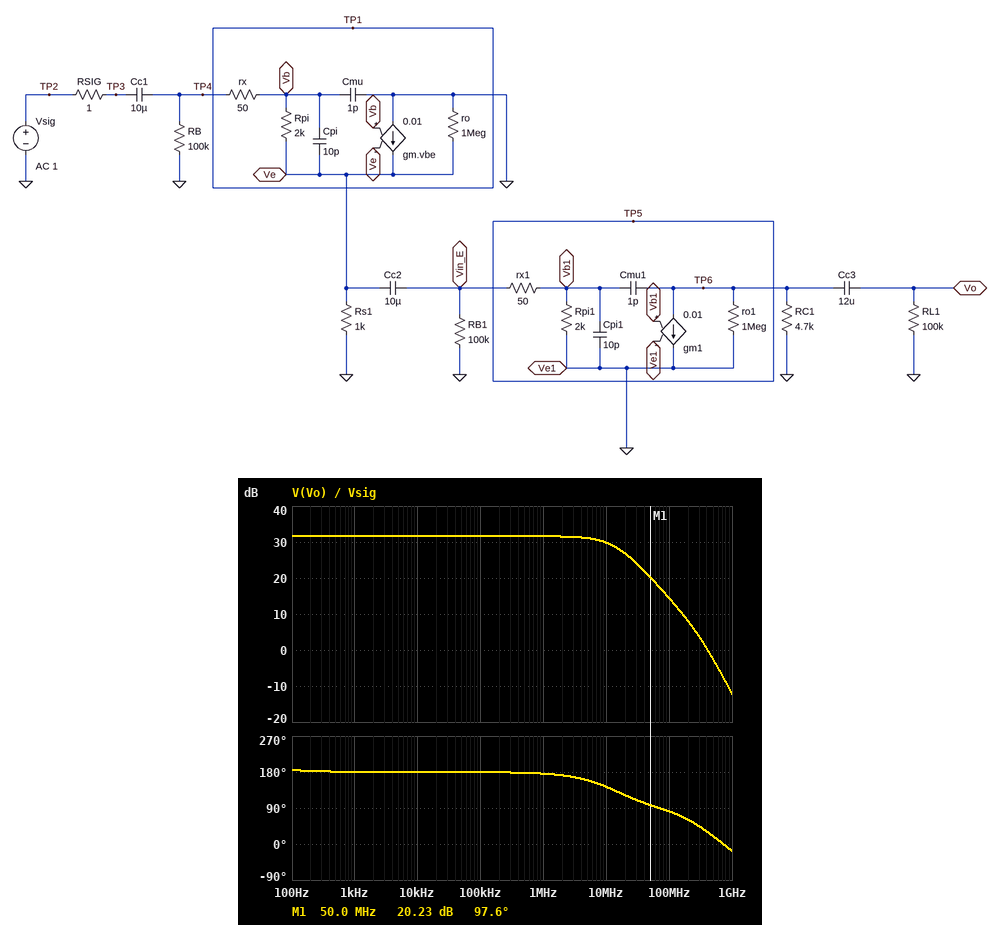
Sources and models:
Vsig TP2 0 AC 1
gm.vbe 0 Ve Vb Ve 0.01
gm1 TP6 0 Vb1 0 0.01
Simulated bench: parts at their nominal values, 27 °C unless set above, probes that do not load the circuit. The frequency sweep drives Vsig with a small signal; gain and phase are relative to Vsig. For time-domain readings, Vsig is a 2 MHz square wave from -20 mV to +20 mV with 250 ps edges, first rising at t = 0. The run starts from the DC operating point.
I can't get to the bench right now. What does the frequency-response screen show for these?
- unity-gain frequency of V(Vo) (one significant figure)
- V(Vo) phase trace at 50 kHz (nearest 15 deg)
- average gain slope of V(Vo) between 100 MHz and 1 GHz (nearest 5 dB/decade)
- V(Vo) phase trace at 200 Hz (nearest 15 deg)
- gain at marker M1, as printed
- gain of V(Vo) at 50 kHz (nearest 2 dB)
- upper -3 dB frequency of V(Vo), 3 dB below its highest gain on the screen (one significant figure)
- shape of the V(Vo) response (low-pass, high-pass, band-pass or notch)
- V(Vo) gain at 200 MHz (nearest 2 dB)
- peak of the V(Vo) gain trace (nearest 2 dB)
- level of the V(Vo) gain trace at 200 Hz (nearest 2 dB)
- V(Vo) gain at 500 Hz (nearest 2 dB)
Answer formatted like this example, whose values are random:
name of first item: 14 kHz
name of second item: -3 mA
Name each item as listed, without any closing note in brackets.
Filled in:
unity-gain frequency of V(Vo): 400 MHz
V(Vo) phase trace at 50 kHz: 180 deg
average gain slope of V(Vo) between 100 MHz and 1 GHz: -25 dB/decade
V(Vo) phase trace at 200 Hz: 180 deg
gain at marker M1, as printed: 20.23 dB
gain of V(Vo) at 50 kHz: 32 dB
upper -3 dB frequency of V(Vo), 3 dB below its highest gain on the screen: 10 MHz
shape of the V(Vo) response: low-pass
V(Vo) gain at 200 MHz: 8 dB
peak of the V(Vo) gain trace: 32 dB
level of the V(Vo) gain trace at 200 Hz: 32 dB
V(Vo) gain at 500 Hz: 32 dB
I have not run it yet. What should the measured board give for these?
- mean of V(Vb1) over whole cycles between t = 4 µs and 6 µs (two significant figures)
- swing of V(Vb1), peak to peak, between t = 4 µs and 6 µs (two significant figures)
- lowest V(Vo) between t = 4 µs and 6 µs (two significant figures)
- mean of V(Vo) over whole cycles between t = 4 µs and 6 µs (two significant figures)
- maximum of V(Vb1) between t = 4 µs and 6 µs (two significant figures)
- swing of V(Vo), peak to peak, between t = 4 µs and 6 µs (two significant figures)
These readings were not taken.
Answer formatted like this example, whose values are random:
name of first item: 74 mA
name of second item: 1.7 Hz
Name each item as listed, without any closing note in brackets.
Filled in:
mean of V(Vb1) over whole cycles between t = 4 µs and 6 µs: 17 mV
swing of V(Vb1), peak to peak, between t = 4 µs and 6 µs: 34 mV
lowest V(Vo) between t = 4 µs and 6 µs: -1.5 V
mean of V(Vo) over whole cycles between t = 4 µs and 6 µs: -760 mV
maximum of V(Vb1) between t = 4 µs and 6 µs: 34 mV
swing of V(Vo), peak to peak, between t = 4 µs and 6 µs: 1.5 V
